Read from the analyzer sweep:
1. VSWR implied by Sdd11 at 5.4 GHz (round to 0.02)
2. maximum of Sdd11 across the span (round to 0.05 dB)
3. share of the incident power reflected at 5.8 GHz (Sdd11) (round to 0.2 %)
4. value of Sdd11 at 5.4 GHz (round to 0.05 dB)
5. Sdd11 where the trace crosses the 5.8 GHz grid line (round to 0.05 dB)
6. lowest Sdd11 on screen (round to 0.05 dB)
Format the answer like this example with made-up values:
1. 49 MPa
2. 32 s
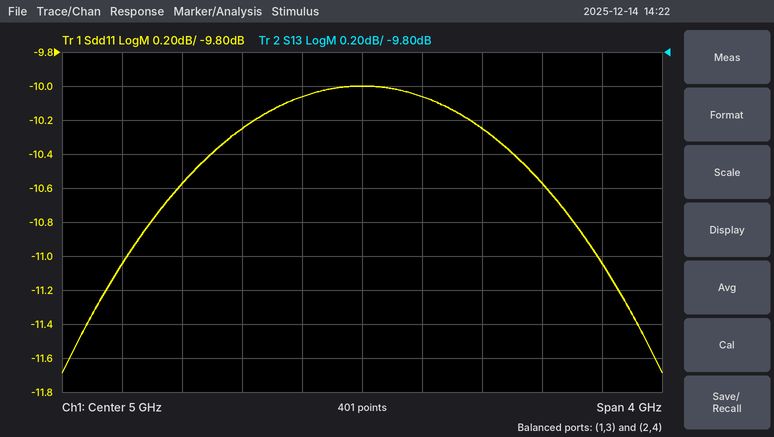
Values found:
1. 1.92
2. -10.00 dB
3. 9.4 %
4. -10.05 dB
5. -10.25 dB
6. -11.70 dB
